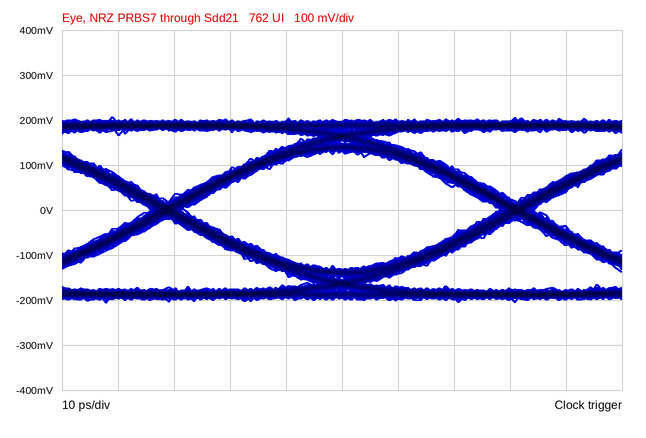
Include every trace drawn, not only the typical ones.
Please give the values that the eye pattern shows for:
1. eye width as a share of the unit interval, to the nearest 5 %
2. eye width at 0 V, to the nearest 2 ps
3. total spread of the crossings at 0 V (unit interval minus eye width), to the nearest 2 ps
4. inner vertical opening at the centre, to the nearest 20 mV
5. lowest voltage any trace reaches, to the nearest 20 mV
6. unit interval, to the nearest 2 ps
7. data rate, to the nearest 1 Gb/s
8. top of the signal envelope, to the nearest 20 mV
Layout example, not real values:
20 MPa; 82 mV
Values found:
90 %; 56 ps; 6 ps; 260 mV; -200 mV; 62 ps; 16 Gb/s; 200 mV
